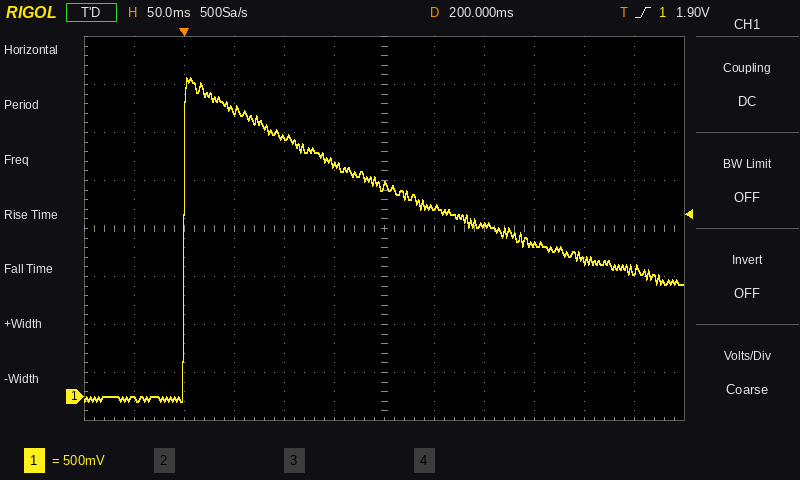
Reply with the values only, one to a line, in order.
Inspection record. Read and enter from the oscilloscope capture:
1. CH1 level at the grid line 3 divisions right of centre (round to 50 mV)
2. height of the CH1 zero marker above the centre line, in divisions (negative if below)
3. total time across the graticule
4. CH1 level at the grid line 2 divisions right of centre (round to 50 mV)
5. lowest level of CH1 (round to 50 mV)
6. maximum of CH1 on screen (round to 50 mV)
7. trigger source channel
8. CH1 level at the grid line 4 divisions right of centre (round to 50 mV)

1.60 V
-3.5 div
600 ms
1.80 V
-50 mV
3.30 V
CH1
1.40 V
